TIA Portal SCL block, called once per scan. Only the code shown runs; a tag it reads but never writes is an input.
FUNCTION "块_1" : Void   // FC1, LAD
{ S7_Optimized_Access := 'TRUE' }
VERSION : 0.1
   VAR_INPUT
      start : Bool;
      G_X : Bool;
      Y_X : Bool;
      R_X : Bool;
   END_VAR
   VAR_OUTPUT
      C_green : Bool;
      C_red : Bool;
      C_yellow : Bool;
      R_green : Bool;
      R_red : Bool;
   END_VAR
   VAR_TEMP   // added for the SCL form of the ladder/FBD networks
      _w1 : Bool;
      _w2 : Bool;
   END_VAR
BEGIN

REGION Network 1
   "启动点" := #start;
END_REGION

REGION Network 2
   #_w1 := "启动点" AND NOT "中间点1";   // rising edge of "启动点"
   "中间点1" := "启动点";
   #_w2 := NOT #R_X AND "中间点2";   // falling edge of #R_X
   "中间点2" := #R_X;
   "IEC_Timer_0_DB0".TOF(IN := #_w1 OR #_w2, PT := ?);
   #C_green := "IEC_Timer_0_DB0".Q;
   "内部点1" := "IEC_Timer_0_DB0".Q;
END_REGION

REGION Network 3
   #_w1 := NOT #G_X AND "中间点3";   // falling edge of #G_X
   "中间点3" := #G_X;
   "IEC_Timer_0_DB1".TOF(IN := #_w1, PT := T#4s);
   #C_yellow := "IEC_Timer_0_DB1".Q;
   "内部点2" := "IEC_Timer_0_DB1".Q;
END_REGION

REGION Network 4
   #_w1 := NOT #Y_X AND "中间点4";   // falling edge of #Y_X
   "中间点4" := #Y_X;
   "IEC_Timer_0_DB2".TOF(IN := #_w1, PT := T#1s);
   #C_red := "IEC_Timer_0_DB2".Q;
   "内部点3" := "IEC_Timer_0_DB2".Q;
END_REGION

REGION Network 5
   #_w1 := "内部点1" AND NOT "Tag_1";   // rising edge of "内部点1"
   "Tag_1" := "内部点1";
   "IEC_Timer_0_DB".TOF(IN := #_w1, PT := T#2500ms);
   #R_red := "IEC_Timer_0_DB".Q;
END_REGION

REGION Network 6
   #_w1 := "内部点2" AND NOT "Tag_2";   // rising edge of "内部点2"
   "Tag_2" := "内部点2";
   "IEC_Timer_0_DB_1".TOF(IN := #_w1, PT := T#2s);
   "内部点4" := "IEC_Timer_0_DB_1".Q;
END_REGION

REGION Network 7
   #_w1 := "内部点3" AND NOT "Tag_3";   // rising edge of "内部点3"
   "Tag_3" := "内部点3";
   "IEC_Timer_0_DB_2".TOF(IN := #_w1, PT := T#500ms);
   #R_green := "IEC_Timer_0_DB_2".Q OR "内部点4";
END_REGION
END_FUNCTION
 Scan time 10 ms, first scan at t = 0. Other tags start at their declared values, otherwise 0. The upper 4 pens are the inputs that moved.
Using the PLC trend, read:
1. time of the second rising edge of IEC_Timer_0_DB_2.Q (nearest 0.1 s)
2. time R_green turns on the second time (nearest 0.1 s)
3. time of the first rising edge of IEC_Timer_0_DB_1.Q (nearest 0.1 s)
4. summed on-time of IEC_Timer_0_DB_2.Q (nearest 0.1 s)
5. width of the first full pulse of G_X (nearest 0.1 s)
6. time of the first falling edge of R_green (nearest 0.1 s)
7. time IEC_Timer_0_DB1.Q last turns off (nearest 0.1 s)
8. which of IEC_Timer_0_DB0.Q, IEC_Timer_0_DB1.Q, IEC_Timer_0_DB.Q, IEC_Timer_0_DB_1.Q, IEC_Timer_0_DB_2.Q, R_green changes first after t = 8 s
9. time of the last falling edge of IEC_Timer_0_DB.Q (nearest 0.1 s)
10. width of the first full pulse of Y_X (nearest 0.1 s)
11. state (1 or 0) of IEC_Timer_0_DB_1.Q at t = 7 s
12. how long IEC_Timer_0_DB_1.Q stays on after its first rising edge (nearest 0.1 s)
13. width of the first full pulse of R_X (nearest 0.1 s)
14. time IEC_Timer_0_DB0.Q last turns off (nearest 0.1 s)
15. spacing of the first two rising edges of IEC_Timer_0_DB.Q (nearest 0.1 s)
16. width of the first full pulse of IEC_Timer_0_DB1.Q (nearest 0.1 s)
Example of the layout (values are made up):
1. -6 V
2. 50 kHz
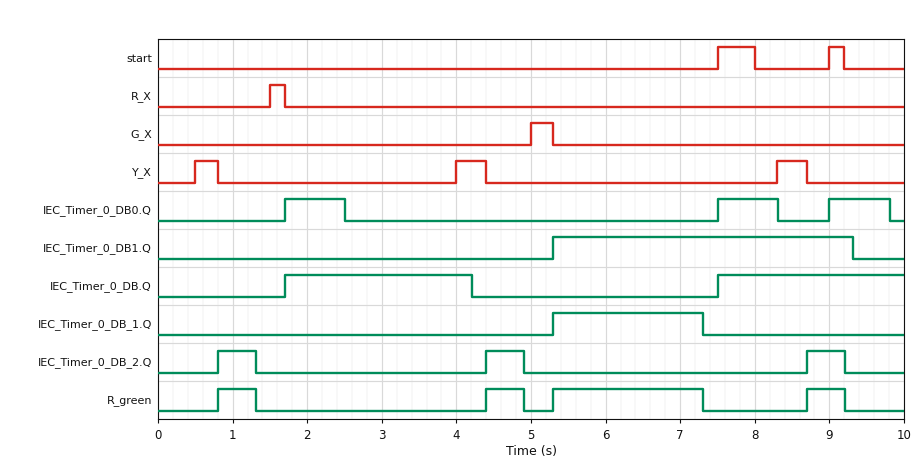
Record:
1. 4.4 s
2. 4.4 s
3. 5.3 s
4. 1.5 s
5. 0.3 s
6. 1.3 s
7. 9.3 s
8. IEC_Timer_0_DB0.Q
9. 4.2 s
10. 0.3 s
11. 1
12. 2.0 s
13. 0.2 s
14. 9.8 s
15. 5.8 s
16. 4.0 s
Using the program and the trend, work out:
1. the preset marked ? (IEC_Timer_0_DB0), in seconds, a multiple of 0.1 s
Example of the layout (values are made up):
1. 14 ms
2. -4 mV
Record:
1. 0.8 s
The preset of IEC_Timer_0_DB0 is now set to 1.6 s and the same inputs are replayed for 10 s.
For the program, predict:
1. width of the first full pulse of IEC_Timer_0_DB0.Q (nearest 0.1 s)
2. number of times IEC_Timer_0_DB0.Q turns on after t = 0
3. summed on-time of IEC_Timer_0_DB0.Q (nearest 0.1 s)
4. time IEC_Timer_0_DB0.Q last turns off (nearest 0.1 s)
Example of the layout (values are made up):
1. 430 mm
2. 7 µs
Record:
1. 1.6 s
2. 2
3. 4.1 s
4. 3.3 s
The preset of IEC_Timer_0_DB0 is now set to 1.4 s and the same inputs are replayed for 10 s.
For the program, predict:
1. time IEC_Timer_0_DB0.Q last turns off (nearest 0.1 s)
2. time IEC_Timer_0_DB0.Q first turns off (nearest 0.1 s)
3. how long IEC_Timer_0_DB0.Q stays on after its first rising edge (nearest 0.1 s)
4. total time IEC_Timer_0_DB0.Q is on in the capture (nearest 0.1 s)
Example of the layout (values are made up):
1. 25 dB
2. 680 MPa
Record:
1. 8.9 s
2. 3.1 s
3. 1.4 s
4. 3.8 s
